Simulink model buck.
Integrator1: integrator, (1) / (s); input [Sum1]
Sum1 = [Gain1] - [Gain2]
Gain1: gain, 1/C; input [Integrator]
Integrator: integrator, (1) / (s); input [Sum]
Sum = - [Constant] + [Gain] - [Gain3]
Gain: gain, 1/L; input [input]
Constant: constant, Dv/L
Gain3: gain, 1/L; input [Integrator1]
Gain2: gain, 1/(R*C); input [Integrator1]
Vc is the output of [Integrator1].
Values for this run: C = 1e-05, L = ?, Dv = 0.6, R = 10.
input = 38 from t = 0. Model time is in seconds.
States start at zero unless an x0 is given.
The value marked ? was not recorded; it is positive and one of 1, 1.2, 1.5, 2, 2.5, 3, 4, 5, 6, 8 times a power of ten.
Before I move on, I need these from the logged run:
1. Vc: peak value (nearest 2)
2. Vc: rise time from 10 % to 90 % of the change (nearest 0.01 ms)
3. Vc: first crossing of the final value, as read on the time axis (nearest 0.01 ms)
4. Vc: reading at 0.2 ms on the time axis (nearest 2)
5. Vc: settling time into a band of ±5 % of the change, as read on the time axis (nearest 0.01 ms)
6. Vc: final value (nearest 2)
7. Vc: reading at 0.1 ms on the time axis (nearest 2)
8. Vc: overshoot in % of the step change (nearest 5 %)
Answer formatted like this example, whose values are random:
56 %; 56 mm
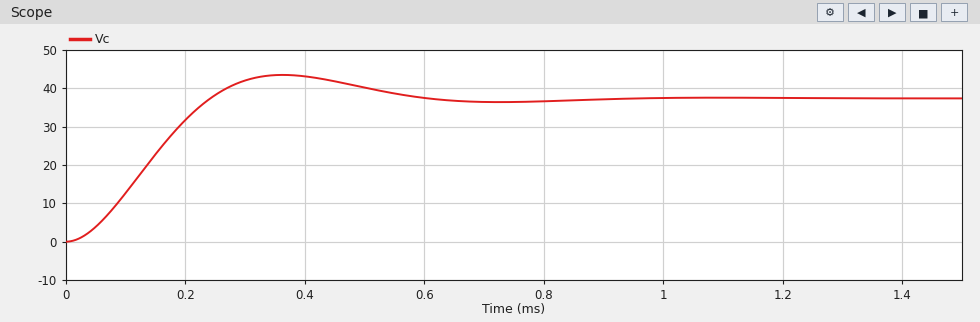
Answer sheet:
44; 0.16 ms; 0.24 ms; 32; 0.53 ms; 38; 12; 15 %
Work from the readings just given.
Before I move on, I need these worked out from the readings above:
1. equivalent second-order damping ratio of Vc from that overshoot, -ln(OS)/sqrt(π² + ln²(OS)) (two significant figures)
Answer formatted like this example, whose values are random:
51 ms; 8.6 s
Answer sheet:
0.52
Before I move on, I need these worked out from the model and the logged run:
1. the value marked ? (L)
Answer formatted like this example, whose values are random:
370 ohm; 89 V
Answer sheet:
0.001
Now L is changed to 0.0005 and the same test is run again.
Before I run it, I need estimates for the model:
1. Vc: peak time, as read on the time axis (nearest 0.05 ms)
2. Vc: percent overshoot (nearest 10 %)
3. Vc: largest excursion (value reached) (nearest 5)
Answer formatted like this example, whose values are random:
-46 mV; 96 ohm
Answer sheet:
0.25 ms; 30 %; 50
